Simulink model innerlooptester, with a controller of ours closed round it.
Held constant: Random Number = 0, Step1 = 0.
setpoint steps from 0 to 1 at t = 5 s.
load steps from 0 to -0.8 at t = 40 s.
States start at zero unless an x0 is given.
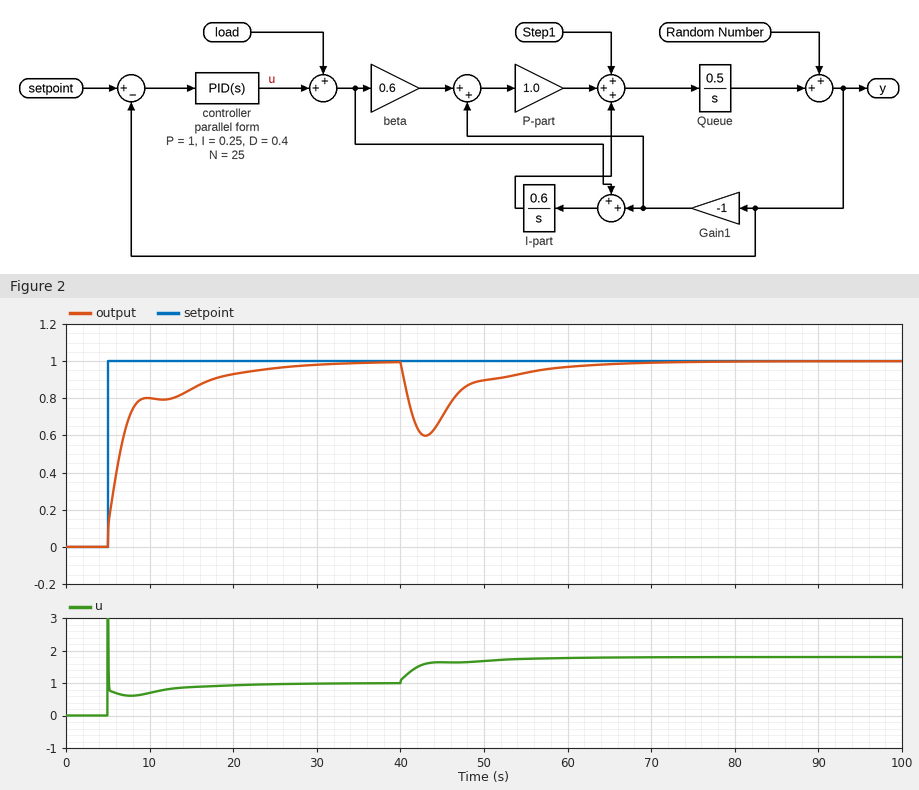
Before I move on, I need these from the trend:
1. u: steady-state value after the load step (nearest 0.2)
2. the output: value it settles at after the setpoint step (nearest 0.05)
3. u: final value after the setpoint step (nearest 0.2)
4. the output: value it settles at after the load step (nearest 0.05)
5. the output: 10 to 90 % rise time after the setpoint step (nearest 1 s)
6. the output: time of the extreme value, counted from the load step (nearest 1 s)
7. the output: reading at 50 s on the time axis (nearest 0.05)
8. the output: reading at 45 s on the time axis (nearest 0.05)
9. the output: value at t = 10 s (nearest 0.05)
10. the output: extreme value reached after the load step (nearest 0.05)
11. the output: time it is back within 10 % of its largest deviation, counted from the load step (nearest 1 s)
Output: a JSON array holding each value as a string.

["1.8", "1.00", "1.0", "1.00", "12 s", "3 s", "0.90", "0.70", "0.80", "0.60", "18 s"]
